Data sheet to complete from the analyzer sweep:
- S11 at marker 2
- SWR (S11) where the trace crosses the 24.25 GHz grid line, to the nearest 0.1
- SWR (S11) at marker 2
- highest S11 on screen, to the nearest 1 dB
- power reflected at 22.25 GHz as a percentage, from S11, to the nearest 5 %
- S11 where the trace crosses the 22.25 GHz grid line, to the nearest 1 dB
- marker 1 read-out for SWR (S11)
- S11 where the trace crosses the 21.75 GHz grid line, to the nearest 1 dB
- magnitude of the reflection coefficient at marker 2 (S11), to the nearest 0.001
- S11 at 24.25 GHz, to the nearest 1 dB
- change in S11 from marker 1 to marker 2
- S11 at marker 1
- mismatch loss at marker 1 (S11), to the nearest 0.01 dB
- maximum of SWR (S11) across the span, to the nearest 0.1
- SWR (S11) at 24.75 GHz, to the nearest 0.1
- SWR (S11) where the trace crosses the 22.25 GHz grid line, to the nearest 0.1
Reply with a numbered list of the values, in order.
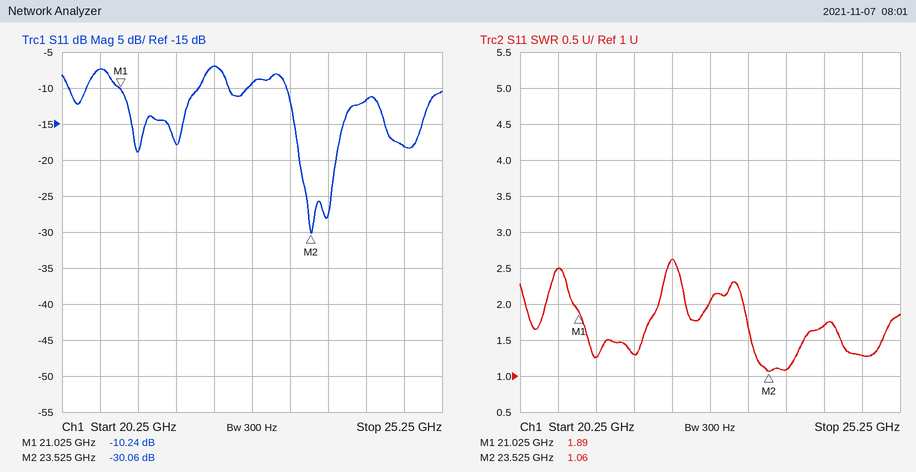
1. -30.06 dB
2. 1.7
3. 1.06
4. -7 dB
5. 20 %
6. -7 dB
7. 1.89
8. -18 dB
9. 0.031
10. -12 dB
11. -19.82 dB
12. -10.24 dB
13. 0.43 dB
14. 2.6
15. 1.3
16. 2.6
